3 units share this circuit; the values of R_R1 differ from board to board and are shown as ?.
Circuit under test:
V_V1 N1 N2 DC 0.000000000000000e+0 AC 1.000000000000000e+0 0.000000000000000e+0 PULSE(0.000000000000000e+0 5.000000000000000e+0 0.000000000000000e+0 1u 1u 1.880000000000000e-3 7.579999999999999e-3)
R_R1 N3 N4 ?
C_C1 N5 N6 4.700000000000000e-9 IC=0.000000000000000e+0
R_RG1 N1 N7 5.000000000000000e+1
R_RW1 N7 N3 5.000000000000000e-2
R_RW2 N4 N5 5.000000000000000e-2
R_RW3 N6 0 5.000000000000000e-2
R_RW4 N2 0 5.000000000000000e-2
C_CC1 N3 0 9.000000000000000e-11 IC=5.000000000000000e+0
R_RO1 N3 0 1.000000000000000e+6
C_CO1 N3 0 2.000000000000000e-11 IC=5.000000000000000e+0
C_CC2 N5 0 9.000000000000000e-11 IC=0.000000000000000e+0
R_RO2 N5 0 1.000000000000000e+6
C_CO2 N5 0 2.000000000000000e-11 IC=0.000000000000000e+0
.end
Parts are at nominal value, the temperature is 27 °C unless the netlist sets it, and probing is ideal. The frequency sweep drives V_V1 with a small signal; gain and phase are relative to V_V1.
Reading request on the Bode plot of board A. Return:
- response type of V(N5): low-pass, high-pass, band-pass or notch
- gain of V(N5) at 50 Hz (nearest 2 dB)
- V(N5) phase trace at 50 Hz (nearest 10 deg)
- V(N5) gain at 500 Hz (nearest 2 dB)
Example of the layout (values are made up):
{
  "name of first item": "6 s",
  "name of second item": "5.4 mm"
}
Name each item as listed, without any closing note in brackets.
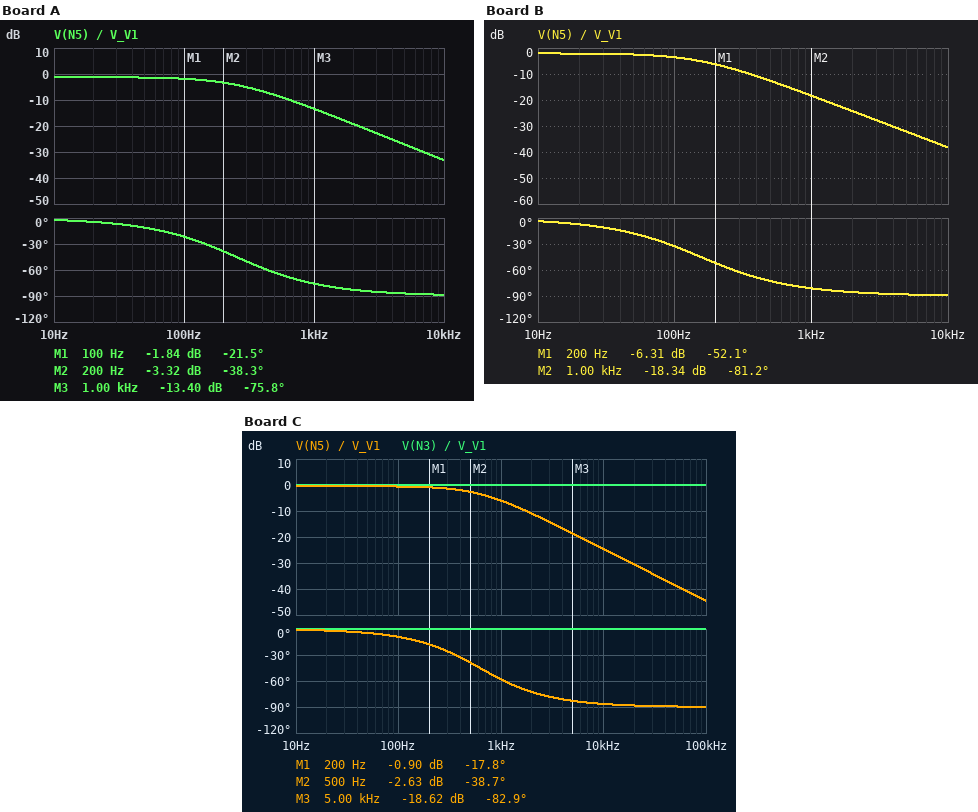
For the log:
{
  "response type of V(N5): low-pass, high-pass, band-pass or notch": "low-pass",
  "gain of V(N5) at 50 Hz": "-2 dB",
  "V(N5) phase trace at 50 Hz": "-10 deg",
  "V(N5) gain at 500 Hz": "-8 dB"
}
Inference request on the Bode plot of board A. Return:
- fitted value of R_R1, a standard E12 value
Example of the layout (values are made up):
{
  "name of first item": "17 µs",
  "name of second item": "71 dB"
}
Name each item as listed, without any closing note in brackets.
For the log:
{
  "fitted value of R_R1, a standard E12 value": "150 kΩ"
}
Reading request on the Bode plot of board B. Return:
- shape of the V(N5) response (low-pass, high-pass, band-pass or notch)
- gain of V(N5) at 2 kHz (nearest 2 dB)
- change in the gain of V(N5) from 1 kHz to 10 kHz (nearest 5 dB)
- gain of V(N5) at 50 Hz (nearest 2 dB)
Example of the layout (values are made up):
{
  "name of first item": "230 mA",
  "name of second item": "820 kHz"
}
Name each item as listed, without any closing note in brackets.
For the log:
{
  "shape of the V(N5) response": "low-pass",
  "gain of V(N5) at 2 kHz": "-24 dB",
  "change in the gain of V(N5) from 1 kHz to 10 kHz": "-20 dB",
  "gain of V(N5) at 50 Hz": "-2 dB"
}
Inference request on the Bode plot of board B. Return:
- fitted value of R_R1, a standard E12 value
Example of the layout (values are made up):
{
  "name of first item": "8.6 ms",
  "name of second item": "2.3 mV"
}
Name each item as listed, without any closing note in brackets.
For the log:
{
  "fitted value of R_R1, a standard E12 value": "270 kΩ"
}
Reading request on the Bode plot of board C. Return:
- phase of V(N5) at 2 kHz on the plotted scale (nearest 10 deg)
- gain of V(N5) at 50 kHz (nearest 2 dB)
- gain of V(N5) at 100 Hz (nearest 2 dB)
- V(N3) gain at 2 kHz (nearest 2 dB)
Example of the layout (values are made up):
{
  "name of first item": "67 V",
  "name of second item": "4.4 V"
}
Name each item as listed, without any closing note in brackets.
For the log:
{
  "phase of V(N5) at 2 kHz on the plotted scale": "-70 deg",
  "gain of V(N5) at 50 kHz": "-38 dB",
  "gain of V(N5) at 100 Hz": "0 dB",
  "V(N3) gain at 2 kHz": "0 dB"
}
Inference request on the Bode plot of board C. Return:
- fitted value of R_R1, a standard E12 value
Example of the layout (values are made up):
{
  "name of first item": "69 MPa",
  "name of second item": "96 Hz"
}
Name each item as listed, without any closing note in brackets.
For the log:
{
  "fitted value of R_R1, a standard E12 value": "56 kΩ"
}
